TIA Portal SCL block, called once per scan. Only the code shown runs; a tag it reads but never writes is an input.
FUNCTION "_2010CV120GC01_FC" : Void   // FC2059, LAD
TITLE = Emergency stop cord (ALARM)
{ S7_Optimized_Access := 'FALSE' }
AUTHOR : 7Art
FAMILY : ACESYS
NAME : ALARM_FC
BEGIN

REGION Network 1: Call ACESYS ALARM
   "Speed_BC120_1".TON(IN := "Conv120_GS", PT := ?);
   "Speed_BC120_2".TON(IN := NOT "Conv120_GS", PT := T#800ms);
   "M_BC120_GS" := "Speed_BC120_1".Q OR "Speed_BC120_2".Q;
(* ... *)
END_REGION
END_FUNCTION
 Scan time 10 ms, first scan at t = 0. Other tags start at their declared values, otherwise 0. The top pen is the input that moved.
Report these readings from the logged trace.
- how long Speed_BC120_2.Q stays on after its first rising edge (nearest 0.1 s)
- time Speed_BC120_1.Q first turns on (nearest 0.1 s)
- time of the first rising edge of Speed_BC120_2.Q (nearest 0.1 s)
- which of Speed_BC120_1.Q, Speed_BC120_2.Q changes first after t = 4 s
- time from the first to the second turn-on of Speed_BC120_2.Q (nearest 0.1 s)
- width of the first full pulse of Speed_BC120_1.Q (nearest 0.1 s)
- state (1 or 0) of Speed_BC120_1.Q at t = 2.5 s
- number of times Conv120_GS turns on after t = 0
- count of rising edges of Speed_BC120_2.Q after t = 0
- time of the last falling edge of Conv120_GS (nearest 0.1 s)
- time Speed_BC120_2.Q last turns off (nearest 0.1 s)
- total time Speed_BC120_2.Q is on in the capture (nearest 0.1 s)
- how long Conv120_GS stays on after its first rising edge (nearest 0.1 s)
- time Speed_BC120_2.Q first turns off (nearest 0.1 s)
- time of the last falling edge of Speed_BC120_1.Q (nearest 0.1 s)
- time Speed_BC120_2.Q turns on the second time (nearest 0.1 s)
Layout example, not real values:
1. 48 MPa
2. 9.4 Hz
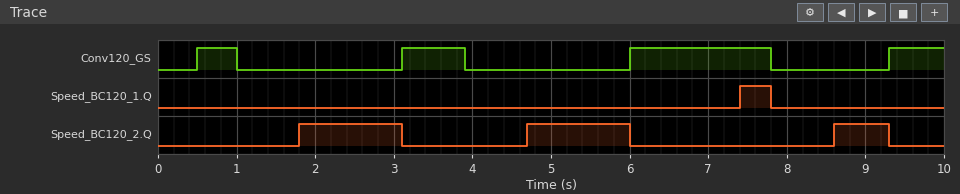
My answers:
1. 1.3 s
2. 7.4 s
3. 1.8 s
4. Speed_BC120_2.Q
5. 2.9 s
6. 0.4 s
7. 0
8. 4
9. 3
10. 7.8 s
11. 9.3 s
12. 3.3 s
13. 0.5 s
14. 3.1 s
15. 7.8 s
16. 4.7 s
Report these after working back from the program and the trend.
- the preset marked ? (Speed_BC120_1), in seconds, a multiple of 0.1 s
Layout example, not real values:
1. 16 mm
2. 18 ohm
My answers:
1. 1.4 s
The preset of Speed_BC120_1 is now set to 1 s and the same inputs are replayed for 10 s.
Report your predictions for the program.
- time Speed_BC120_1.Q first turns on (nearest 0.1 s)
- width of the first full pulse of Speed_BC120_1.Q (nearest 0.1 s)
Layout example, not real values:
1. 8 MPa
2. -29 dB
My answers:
1. 7.0 s
2. 0.8 s
